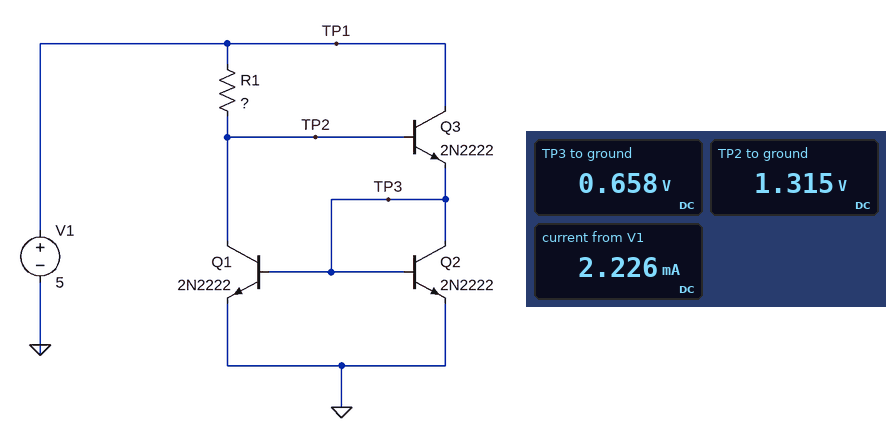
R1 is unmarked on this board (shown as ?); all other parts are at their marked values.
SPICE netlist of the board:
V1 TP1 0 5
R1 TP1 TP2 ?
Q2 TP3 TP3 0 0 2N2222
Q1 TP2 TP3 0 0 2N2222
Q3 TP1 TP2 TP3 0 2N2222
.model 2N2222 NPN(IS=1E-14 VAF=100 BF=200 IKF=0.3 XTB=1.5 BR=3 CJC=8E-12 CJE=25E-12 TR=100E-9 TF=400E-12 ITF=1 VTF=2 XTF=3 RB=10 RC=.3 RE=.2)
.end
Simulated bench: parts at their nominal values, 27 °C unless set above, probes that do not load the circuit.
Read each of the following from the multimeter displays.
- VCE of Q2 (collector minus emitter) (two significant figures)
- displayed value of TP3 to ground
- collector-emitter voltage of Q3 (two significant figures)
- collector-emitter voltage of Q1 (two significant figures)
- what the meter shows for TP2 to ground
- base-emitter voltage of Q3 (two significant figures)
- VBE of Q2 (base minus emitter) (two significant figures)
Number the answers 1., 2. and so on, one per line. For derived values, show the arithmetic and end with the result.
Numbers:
1. 658 mV = 660 mV
2. 0.658 V
3. 5 V - 658 mV = 4.3 V
4. 1.315 V = 1.3 V
5. 1.315 V
6. 1.315 V - 658 mV = 660 mV
7. 658 mV = 660 mV
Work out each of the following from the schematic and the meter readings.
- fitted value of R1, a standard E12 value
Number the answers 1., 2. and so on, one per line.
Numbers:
1. 3.3 kΩ
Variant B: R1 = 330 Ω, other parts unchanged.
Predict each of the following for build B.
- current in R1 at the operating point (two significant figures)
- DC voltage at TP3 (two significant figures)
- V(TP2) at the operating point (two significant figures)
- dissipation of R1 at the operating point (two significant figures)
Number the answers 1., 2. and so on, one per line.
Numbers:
1. 11 mA
2. 720 mV
3. 1.4 V
4. 38 mW
